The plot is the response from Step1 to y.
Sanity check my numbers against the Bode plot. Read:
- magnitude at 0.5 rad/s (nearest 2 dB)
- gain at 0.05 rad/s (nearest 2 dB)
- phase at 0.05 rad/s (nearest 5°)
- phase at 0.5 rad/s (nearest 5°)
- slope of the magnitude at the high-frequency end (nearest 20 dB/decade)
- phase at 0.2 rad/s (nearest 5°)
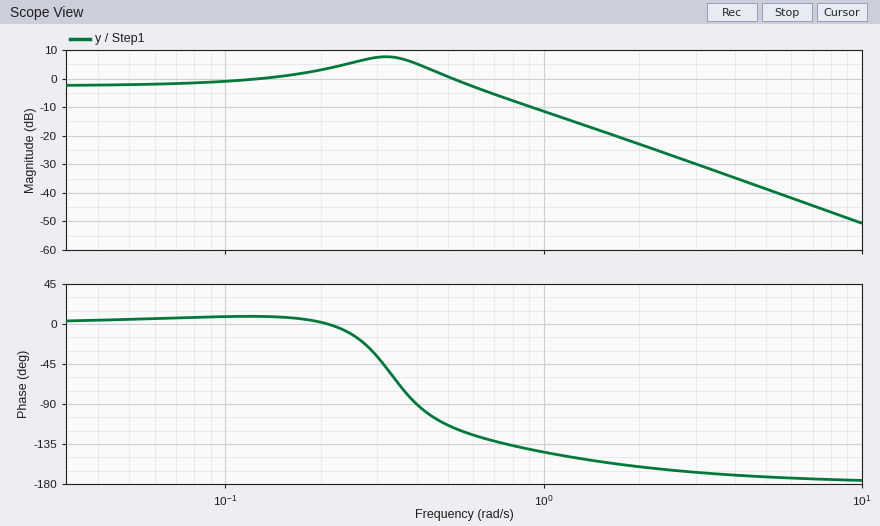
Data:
0 dB
-2 dB
5°
-115°
-40 dB/decade
0°
